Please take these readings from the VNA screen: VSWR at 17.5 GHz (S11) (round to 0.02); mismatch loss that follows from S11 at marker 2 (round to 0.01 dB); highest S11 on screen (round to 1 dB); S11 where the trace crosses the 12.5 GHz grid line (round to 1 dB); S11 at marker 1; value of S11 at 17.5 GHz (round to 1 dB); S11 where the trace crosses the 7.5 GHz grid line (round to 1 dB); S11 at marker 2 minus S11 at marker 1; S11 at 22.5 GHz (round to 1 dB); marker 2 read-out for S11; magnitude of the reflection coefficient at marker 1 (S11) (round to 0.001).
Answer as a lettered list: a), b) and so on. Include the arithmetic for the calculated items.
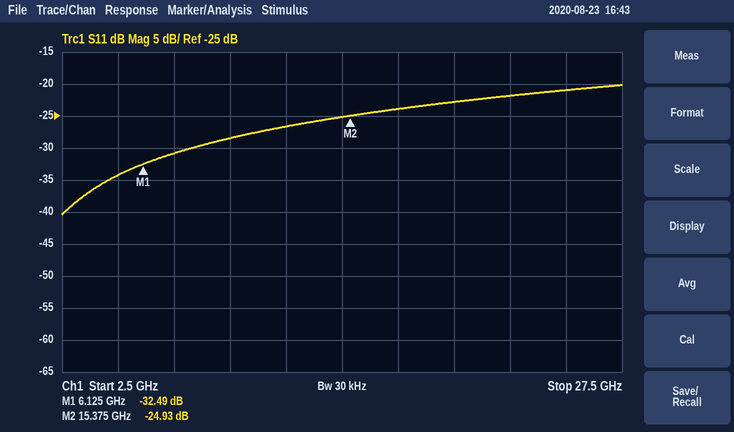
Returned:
a) |Γ| = 10^(-24/20) = 0.0631; VSWR = (1 + 0.0631)/(1 − 0.0631) ≈ 1.13, so 1.14 to the nearest 0.02
b) −10 log10(1 − 10^(-24.93/10)) ≈ 0.01 dB
c) -20 dB
d) -27 dB
e) -32.49 dB
f) -24 dB
g) -31 dB
h) -24.93 − (-32.49) = 7.56 dB
i) -22 dB
j) -24.93 dB
k) 10^(-32.49/20) ≈ 0.024
